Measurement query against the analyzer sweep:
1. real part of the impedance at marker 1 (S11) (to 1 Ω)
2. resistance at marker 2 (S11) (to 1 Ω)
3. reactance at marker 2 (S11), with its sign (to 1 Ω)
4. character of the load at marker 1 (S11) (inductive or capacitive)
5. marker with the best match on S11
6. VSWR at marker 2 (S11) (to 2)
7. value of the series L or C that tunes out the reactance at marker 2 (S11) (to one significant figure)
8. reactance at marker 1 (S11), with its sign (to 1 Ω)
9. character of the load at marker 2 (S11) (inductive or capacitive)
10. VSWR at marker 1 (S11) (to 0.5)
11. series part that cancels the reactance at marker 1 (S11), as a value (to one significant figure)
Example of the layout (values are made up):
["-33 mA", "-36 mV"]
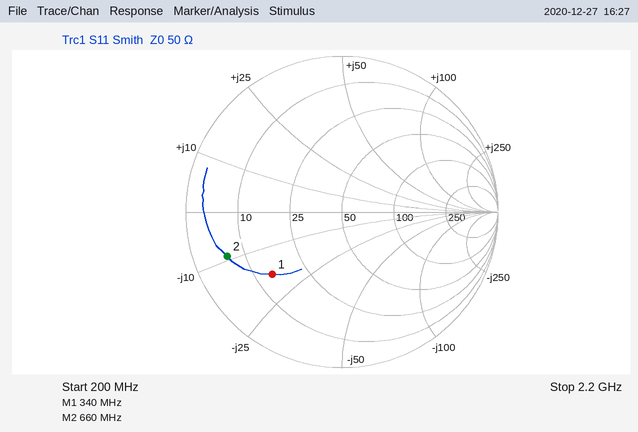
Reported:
["14 Ω", "6 Ω", "-9 Ω", "capacitive", "marker 1", "8", "2 nH", "-18 Ω", "capacitive", "4.0", "8 nH"]
